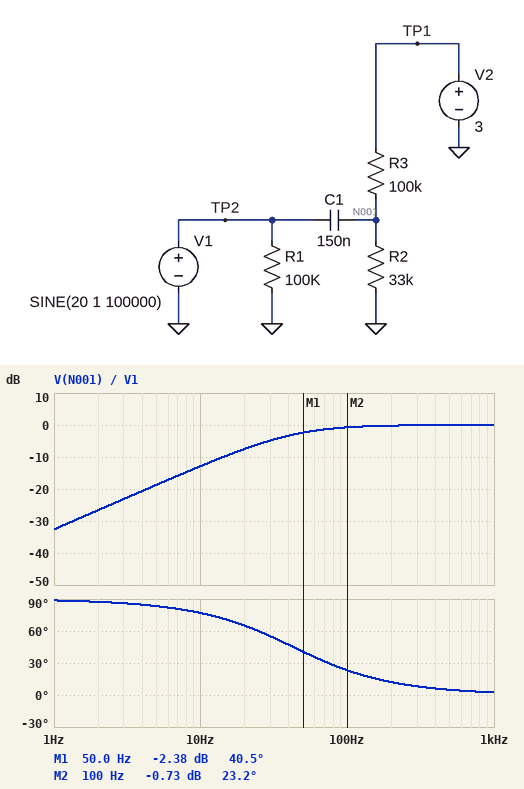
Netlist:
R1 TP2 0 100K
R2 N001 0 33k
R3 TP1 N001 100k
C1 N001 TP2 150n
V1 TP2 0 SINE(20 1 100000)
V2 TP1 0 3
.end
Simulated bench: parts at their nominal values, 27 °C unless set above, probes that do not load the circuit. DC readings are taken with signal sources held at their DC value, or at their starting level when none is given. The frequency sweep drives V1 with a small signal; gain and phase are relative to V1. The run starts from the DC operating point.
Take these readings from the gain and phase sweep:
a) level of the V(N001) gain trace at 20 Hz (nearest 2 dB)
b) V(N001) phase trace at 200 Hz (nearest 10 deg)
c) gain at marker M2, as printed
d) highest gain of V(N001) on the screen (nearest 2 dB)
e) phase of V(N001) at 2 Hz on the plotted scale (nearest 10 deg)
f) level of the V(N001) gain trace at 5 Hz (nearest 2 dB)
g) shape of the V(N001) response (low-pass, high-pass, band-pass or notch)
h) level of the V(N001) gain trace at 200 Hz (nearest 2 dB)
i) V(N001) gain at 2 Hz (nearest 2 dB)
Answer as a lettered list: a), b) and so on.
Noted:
a) -8 dB
b) 10 deg
c) -0.73 dB
d) 0 dB
e) 90 deg
f) -18 dB
g) high-pass
h) 0 dB
i) -26 dB
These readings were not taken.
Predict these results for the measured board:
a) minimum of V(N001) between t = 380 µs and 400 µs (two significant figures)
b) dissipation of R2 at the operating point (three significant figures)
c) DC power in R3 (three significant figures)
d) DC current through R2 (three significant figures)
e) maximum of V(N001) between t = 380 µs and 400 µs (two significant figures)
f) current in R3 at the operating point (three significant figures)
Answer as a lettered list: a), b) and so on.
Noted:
a) -260 mV
b) 16.8 µW
c) 50.9 µW
d) 22.6 µA
e) 1.7 V
f) 22.6 µA
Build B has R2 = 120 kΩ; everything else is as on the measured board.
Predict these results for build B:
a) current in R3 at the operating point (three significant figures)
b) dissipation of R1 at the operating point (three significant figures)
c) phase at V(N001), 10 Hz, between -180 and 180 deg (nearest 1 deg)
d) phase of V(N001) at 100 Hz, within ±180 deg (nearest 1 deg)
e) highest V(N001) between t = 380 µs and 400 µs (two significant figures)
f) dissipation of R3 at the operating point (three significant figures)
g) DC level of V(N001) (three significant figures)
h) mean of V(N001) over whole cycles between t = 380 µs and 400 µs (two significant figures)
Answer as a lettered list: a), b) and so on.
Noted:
a) 13.6 µA
b) 4.00 mW
c) 63 deg
d) 11 deg
e) 2.6 V
f) 18.6 µW
g) 1.64 V
h) 1.6 V
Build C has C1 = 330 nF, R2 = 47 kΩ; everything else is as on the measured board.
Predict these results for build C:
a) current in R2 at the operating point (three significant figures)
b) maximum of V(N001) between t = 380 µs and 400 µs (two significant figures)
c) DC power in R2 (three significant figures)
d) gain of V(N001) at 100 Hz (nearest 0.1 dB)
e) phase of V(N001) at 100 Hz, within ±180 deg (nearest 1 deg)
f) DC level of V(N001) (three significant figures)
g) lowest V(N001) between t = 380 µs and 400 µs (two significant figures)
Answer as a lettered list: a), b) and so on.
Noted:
a) 20.4 µA
b) 2.0 V
c) 19.6 µW
d) -0.1 dB
e) 9 deg
f) 959 mV
g) -41 mV
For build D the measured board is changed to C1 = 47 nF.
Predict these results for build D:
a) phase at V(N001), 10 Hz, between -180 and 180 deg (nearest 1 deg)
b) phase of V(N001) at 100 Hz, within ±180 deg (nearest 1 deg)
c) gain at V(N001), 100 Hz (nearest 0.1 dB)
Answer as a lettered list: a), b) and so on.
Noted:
a) 86 deg
b) 54 deg
c) -4.6 dB
